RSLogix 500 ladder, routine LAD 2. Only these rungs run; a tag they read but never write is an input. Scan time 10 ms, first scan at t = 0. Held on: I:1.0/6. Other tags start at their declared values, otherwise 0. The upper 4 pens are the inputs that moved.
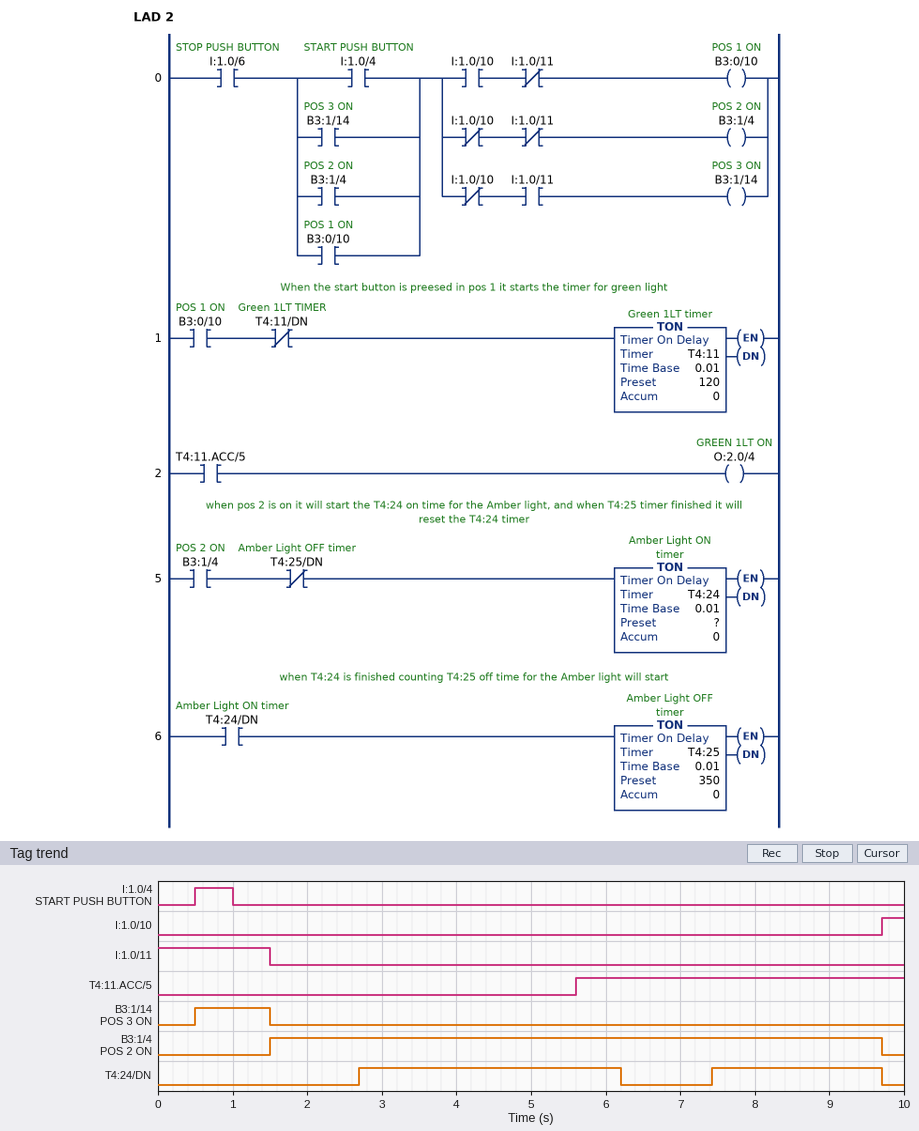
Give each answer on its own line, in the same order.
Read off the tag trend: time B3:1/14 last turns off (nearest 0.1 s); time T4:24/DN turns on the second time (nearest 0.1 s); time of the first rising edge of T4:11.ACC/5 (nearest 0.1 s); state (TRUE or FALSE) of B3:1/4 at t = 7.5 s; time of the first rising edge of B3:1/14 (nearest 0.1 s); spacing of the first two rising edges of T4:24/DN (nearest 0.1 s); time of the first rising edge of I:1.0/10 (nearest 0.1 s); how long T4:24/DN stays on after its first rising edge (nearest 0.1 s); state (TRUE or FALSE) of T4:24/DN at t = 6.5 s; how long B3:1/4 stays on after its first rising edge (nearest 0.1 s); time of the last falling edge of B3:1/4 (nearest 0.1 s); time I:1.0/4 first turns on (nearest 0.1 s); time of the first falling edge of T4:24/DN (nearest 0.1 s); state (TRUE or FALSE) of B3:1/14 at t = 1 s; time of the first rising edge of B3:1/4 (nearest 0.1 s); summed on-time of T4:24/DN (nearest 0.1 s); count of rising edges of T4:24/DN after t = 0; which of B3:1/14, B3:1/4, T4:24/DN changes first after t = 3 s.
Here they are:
1.5 s
7.4 s
5.6 s
TRUE
0.5 s
4.7 s
9.7 s
3.5 s
FALSE
8.2 s
9.7 s
0.5 s
6.2 s
TRUE
1.5 s
5.8 s
2
T4:24/DN
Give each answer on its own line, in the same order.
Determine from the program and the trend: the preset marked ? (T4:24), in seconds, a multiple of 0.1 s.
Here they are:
1.2 s
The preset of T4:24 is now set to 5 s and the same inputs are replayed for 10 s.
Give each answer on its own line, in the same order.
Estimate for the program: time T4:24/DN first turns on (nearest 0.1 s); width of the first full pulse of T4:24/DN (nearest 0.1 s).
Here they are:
6.5 s
3.2 s
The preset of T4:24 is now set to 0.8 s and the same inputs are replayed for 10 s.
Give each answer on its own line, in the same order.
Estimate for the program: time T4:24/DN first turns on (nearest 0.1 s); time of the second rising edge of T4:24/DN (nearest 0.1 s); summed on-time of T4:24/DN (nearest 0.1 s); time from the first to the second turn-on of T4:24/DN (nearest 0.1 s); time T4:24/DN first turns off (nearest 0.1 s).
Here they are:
2.3 s
6.6 s
6.6 s
4.3 s
5.8 s
